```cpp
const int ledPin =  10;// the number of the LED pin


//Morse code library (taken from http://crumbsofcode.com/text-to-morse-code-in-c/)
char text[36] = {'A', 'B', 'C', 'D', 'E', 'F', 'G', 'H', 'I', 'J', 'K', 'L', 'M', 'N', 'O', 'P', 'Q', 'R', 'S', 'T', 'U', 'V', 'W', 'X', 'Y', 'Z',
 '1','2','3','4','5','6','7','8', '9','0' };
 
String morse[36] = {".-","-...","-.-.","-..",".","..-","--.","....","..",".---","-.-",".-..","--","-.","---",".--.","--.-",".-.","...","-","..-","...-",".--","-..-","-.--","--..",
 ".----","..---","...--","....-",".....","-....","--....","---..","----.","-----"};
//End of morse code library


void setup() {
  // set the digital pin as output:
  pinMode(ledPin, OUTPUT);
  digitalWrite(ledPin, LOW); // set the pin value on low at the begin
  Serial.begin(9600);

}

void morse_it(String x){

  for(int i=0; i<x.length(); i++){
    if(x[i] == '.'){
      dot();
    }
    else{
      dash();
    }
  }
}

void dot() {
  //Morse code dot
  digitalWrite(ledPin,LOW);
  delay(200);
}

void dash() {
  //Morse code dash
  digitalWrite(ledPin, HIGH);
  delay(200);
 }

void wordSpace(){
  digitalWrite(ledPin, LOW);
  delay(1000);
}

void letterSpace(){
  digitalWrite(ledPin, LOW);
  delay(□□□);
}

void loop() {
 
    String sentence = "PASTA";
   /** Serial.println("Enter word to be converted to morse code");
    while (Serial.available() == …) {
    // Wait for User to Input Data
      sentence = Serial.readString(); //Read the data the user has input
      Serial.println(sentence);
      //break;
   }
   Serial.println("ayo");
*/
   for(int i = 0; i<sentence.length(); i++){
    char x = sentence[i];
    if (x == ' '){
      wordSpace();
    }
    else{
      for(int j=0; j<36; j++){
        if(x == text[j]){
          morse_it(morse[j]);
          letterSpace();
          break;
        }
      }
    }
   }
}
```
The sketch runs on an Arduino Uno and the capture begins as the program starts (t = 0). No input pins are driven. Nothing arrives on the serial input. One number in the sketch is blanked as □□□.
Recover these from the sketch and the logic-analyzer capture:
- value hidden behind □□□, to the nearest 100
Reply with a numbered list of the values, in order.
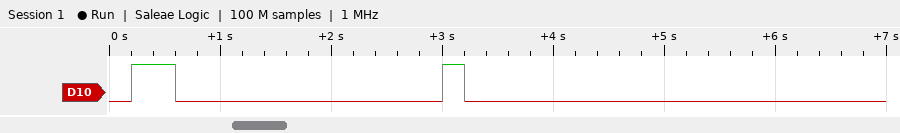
1. 2000
